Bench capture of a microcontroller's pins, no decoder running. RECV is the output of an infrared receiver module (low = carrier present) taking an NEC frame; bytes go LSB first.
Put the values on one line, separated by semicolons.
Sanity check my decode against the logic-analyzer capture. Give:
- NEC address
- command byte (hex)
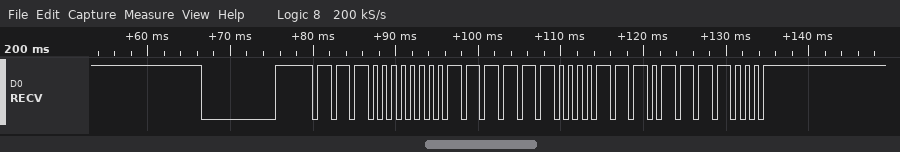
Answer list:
0x07; 0xE1
